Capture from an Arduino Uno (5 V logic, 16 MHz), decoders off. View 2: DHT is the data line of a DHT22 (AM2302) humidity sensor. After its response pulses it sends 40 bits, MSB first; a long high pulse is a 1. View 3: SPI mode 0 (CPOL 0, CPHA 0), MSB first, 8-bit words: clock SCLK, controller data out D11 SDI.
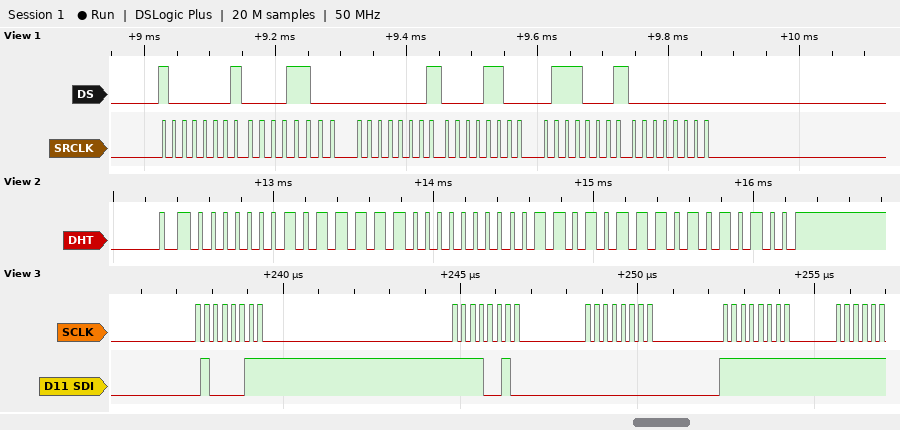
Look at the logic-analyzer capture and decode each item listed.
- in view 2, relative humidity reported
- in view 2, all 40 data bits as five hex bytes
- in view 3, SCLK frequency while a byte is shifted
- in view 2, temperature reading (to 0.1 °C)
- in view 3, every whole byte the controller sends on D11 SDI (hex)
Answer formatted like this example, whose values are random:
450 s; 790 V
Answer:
38.0 %; 01 7C 00 D7 54; 4 MHz; 21.5 °C; 0x43 0xF2 0x00 0xFF
